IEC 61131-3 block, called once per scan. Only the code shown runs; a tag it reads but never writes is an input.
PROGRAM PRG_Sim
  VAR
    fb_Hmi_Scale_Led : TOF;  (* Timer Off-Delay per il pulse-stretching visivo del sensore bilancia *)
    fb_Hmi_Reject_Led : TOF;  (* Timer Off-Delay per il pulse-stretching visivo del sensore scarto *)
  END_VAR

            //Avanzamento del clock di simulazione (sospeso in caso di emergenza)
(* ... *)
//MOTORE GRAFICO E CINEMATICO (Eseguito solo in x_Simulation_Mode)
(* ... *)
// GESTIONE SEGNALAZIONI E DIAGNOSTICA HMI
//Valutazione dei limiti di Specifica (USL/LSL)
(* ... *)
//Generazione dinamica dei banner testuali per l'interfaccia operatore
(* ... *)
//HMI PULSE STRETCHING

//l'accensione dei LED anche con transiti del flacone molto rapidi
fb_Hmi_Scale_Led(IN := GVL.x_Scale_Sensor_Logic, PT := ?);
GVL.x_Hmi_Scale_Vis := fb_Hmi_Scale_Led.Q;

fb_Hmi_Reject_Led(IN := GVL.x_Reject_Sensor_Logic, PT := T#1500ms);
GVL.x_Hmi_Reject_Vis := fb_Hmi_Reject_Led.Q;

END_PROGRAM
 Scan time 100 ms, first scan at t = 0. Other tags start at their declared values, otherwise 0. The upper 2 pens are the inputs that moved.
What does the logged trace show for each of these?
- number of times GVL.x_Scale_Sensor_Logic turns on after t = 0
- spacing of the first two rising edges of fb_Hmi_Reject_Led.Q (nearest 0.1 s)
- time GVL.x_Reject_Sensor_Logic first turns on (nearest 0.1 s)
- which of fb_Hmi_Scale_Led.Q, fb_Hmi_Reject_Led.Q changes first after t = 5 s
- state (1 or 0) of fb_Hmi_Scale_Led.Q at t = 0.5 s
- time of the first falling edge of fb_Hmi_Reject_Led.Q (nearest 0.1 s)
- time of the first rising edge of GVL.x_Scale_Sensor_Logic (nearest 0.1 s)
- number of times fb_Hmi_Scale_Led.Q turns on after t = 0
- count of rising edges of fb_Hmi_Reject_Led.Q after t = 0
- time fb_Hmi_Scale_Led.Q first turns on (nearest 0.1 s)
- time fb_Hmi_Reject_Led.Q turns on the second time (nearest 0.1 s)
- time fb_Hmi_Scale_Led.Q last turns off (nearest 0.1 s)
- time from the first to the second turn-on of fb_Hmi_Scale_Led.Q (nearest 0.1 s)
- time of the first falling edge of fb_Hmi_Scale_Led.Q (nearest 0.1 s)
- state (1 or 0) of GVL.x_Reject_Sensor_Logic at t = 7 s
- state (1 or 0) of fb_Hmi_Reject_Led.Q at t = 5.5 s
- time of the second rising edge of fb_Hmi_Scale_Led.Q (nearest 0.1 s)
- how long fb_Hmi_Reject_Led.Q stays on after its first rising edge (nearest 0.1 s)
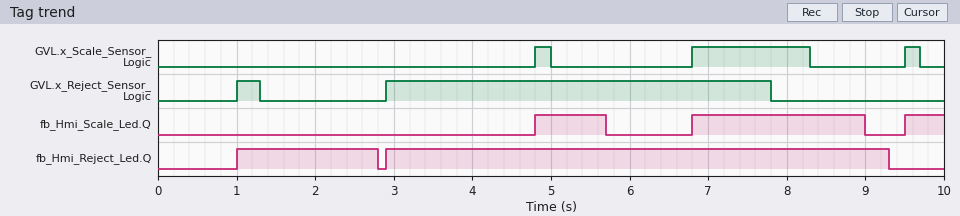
3
1.9 s
1.0 s
fb_Hmi_Scale_Led.Q
0
2.8 s
4.8 s
3
2
4.8 s
2.9 s
9.0 s
2.0 s
5.7 s
1
1
6.8 s
1.8 s
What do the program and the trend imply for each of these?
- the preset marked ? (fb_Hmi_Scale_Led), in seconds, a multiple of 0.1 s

0.7 s
